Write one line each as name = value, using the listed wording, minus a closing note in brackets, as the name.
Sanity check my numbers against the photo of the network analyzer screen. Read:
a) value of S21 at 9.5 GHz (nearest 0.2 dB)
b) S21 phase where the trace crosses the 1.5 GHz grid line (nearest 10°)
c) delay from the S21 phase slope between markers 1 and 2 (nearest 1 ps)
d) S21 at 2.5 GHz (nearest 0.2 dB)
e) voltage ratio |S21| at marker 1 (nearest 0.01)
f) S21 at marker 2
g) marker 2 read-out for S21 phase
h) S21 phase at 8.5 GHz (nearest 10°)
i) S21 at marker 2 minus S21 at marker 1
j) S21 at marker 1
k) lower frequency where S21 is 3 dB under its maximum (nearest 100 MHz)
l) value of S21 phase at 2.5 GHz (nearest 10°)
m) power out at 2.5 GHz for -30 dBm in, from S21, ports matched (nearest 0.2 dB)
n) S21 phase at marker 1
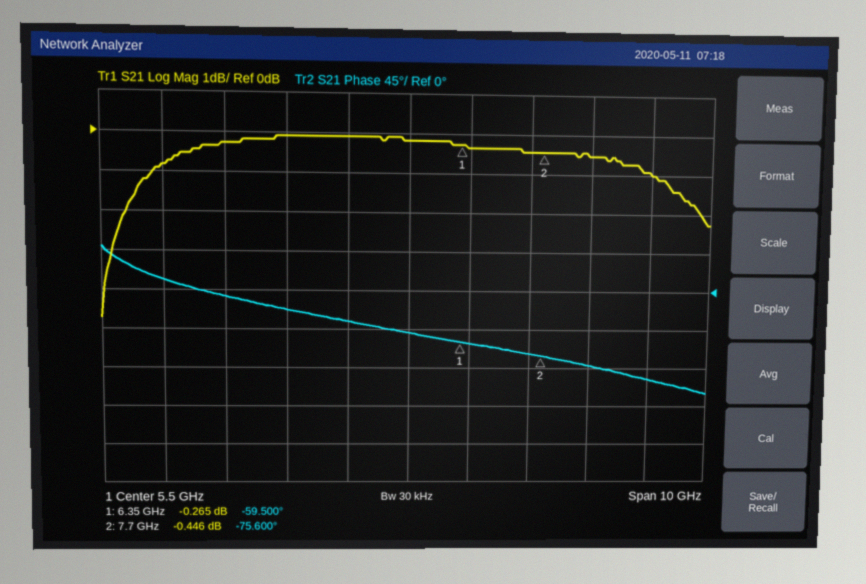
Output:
value of S21 at 9.5 GHz = -1.0 dB
S21 phase where the trace crosses the 1.5 GHz grid line = 10°
delay from the S21 phase slope between markers 1 and 2 = 33 ps
S21 at 2.5 GHz = -0.2 dB
voltage ratio |S21| at marker 1 = 0.97
S21 at marker 2 = -0.446 dB
marker 2 read-out for S21 phase = -75.600°
S21 phase at 8.5 GHz = -90°
S21 at marker 2 minus S21 at marker 1 = -0.181 dB
S21 at marker 1 = -0.265 dB
lower frequency where S21 is 3 dB under its maximum = 700 MHz
value of S21 phase at 2.5 GHz = -10°
power out at 2.5 GHz for -30 dBm in, from S21, ports matched = -30.2 dBm
S21 phase at marker 1 = -59.500°
